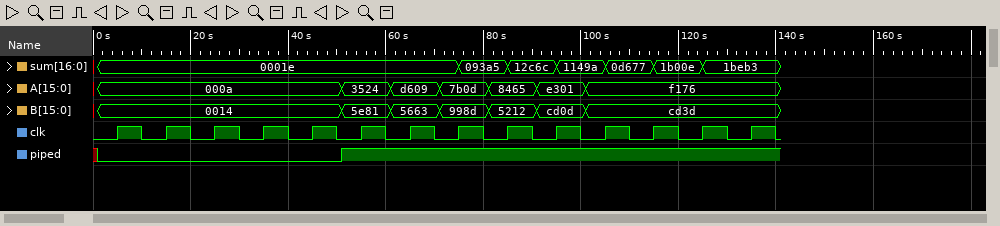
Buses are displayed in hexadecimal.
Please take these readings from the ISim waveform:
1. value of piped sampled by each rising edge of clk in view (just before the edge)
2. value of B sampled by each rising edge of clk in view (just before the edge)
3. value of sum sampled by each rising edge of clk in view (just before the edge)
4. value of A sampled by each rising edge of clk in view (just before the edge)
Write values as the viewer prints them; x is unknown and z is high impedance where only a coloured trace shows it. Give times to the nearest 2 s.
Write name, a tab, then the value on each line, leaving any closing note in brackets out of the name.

value of piped sampled by each rising edge of clk in view	0 0 0 0 0 1 1 1 1 1 1 1 1 1
value of B sampled by each rising edge of clk in view	0014, 0014, 0014, 0014, 0014, 5e81, 5663, 998d, 5212, cd0d, cd3d, cd3d, cd3d, cd3d
value of sum sampled by each rising edge of clk in view	0001e, 0001e, 0001e, 0001e, 0001e, 0001e, 0001e, 0001e, 093a5, 12c6c, 1149a, 0d677, 1b00e, 1beb3
value of A sampled by each rising edge of clk in view	000a, 000a, 000a, 000a, 000a, 3524, d609, 7b0d, 8465, e301, f176, f176, f176, f176
